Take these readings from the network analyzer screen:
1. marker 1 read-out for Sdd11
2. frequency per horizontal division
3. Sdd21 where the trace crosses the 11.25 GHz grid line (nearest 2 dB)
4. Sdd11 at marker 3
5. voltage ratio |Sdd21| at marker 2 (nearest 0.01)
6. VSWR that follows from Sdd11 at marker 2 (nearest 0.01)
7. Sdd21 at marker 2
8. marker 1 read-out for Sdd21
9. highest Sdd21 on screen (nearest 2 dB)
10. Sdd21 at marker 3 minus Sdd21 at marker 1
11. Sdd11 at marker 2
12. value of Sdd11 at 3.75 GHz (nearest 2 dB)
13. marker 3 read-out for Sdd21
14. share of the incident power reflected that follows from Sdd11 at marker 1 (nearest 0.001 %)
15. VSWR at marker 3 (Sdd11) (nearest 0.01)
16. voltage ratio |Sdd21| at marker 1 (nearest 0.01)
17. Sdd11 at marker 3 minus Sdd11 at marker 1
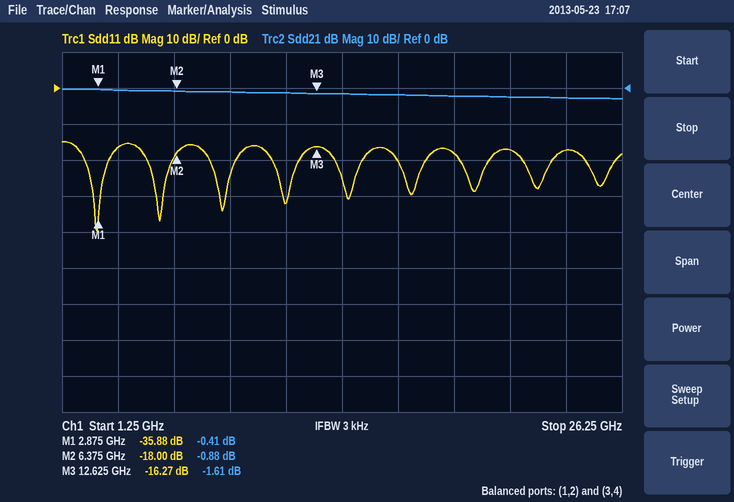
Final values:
-35.88 dB
2.5 GHz
-2 dB
-16.27 dB
0.90
1.29
-0.88 dB
-0.41 dB
0 dB
-1.20 dB
-18.00 dB
-16 dB
-1.61 dB
0.026 %
1.36
0.95
19.61 dB
